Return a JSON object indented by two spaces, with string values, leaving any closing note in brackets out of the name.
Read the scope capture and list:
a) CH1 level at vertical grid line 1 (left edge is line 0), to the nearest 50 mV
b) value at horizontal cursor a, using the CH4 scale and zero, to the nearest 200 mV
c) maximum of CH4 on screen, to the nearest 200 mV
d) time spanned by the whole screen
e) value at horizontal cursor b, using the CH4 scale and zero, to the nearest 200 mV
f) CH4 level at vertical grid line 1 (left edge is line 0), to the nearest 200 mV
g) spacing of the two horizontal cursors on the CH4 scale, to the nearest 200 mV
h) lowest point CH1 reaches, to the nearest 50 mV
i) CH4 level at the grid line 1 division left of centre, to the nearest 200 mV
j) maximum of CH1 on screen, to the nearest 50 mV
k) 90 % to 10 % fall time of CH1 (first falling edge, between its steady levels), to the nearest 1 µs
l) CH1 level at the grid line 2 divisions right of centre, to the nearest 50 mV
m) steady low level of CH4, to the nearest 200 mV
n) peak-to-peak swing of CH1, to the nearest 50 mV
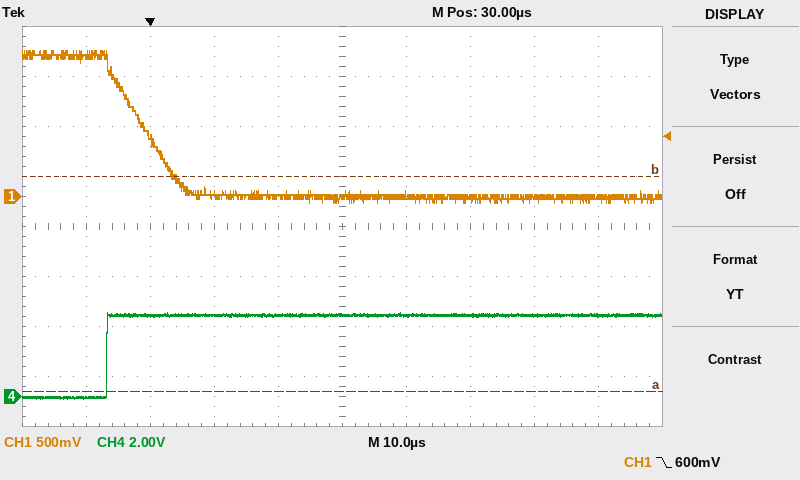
{
  "CH1 level at vertical grid line 1 (left edge is line 0), to the nearest 50 mV": "1.40 V",
  "value at horizontal cursor a, using the CH4 scale and zero, to the nearest 200 mV": "200 mV",
  "maximum of CH4 on screen, to the nearest 200 mV": "3.4 V",
  "time spanned by the whole screen": "100 µs",
  "value at horizontal cursor b, using the CH4 scale and zero, to the nearest 200 mV": "8.8 V",
  "CH4 level at vertical grid line 1 (left edge is line 0), to the nearest 200 mV": "0.0 V",
  "spacing of the two horizontal cursors on the CH4 scale, to the nearest 200 mV": "8.6 V",
  "lowest point CH1 reaches, to the nearest 50 mV": "-50 mV",
  "CH4 level at the grid line 1 division left of centre, to the nearest 200 mV": "3.2 V",
  "maximum of CH1 on screen, to the nearest 50 mV": "1.45 V",
  "90 % to 10 % fall time of CH1 (first falling edge, between its steady levels), to the nearest 1 µs": "11 µs",
  "CH1 level at the grid line 2 divisions right of centre, to the nearest 50 mV": "0 mV",
  "steady low level of CH4, to the nearest 200 mV": "0.0 V",
  "peak-to-peak swing of CH1, to the nearest 50 mV": "1.50 V"
}
